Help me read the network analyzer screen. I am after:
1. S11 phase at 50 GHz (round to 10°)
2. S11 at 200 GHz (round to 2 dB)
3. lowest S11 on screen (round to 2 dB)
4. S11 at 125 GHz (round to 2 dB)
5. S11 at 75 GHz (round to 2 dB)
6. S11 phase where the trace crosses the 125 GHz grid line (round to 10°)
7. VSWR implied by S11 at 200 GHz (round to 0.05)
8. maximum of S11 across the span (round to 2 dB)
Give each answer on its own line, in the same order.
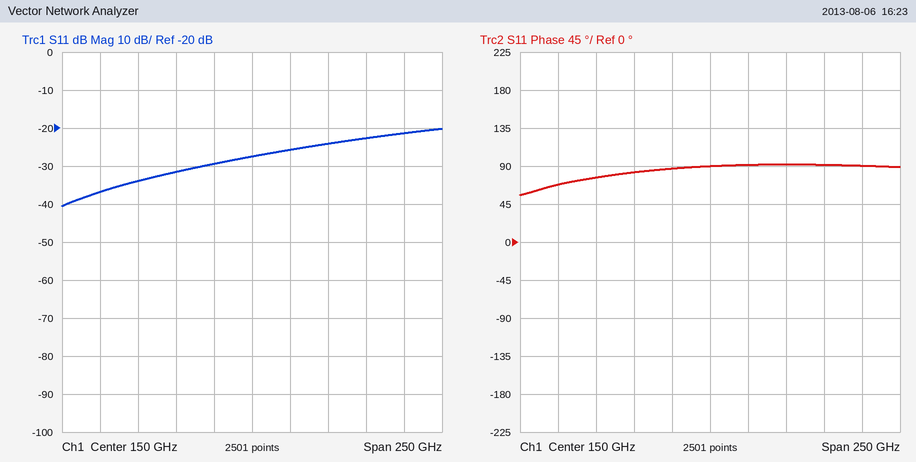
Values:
70°
-24 dB
-40 dB
-30 dB
-34 dB
90°
1.15
-20 dB
